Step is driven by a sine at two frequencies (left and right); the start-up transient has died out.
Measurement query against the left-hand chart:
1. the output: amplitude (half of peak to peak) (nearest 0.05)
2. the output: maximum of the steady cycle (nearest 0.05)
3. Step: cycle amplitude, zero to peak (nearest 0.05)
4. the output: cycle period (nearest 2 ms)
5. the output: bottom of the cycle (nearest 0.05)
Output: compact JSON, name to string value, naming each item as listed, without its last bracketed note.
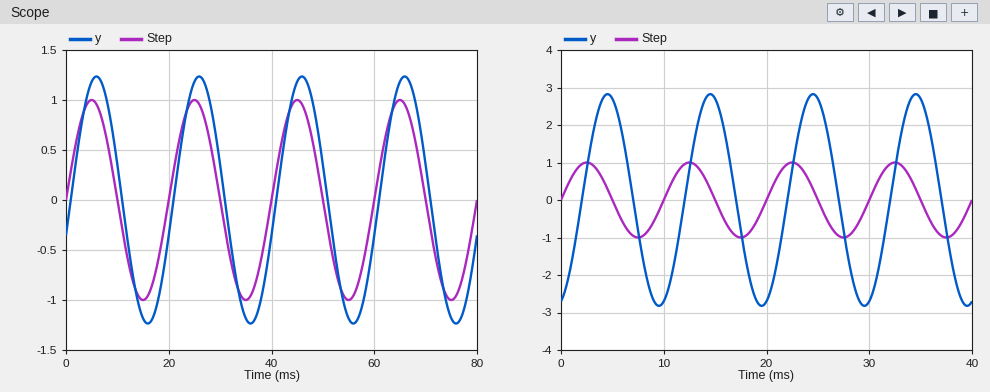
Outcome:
{"the output: amplitude (half of peak to peak)": "1.25", "the output: maximum of the steady cycle": "1.25", "Step: cycle amplitude, zero to peak": "1.00", "the output: cycle period": "20 ms", "the output: bottom of the cycle": "-1.25"}
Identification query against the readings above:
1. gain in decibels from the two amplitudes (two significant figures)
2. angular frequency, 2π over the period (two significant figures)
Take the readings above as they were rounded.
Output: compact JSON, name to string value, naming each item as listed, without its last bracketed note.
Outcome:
{"gain in decibels from the two amplitudes": "1.9 dB", "angular frequency, 2π over the period": "0.31 rad/ms"}
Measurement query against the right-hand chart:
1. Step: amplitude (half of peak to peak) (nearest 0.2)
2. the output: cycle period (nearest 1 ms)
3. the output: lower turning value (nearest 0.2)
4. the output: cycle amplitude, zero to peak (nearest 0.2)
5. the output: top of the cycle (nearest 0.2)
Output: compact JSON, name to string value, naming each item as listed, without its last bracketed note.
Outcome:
{"Step: amplitude (half of peak to peak)": "1.0", "the output: cycle period": "10 ms", "the output: lower turning value": "-2.8", "the output: cycle amplitude, zero to peak": "2.8", "the output: top of the cycle": "2.8"}
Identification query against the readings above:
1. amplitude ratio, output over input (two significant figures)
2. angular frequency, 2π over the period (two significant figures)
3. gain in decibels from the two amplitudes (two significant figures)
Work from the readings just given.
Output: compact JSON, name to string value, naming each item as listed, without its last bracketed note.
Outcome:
{"amplitude ratio, output over input": "2.8", "angular frequency, 2π over the period": "0.63 rad/ms", "gain in decibels from the two amplitudes": "8.9 dB"}
